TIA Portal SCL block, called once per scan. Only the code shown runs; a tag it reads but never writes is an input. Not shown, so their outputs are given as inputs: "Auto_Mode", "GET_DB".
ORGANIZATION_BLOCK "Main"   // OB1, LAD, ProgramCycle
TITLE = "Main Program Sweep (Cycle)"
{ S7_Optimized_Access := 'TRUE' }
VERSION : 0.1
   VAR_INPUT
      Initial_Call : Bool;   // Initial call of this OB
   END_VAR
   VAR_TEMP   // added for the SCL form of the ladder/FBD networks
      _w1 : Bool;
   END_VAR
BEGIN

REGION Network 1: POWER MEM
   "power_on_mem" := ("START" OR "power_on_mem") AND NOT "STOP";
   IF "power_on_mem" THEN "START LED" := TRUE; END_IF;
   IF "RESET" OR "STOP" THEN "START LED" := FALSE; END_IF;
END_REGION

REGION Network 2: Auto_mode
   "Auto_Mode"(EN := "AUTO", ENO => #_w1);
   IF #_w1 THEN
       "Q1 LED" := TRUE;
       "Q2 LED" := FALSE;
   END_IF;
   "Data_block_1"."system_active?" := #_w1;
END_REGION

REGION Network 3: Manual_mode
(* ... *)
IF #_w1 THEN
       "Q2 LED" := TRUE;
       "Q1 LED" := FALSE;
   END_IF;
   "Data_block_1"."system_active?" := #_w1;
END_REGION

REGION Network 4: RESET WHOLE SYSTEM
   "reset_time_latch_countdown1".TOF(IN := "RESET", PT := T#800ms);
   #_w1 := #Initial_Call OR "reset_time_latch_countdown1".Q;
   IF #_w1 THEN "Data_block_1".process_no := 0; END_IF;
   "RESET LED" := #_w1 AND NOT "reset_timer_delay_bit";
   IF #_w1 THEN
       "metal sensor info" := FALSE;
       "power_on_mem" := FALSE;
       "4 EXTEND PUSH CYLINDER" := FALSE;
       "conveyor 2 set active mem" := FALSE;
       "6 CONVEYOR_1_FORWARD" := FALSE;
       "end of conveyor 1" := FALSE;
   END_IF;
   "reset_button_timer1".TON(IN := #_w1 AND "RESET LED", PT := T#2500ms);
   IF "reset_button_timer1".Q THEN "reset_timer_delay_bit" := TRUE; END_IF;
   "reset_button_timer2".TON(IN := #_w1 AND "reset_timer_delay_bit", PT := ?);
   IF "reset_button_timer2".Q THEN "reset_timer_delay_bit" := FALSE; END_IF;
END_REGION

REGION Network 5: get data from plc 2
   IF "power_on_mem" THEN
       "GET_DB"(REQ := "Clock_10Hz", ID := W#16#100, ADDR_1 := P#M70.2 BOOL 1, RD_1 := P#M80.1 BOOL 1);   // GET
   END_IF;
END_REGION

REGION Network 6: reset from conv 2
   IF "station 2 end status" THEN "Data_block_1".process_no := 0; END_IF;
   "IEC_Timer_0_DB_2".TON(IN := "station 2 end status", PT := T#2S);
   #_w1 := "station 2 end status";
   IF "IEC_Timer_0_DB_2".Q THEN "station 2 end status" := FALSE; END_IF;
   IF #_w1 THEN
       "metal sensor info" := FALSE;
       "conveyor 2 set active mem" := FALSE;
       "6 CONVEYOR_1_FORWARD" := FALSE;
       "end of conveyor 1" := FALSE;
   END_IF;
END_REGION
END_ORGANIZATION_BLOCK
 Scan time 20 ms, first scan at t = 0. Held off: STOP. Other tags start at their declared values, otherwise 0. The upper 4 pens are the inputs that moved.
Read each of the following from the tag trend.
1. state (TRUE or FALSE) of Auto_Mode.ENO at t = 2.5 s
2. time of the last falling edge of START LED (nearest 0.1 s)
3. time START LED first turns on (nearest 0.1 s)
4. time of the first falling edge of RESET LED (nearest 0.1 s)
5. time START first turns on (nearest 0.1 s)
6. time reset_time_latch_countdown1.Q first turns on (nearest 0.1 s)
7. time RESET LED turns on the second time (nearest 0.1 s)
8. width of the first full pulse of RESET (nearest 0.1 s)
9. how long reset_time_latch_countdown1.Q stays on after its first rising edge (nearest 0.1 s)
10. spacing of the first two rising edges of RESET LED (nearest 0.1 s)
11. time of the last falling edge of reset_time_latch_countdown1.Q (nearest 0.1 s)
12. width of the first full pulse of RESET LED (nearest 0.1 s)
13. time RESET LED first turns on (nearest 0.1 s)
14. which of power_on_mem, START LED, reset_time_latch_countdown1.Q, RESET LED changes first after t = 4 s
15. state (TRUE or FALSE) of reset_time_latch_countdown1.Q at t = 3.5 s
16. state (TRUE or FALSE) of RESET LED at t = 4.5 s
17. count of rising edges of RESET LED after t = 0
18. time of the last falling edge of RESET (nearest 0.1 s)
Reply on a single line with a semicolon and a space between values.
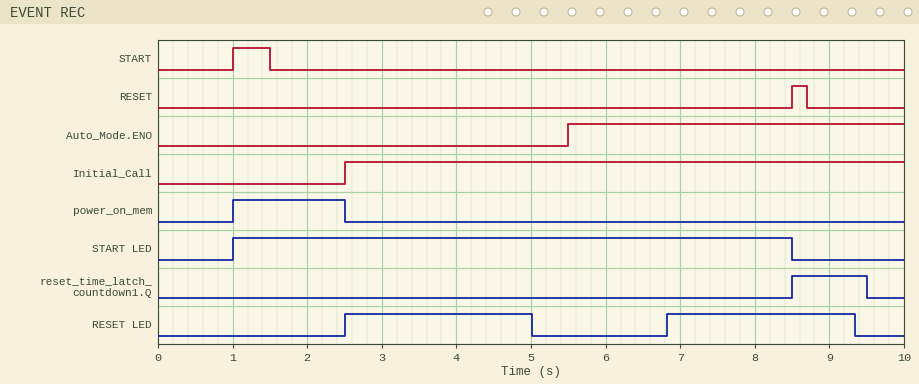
FALSE; 8.5 s; 1.0 s; 5.0 s; 1.0 s; 8.5 s; 6.8 s; 0.2 s; 1.0 s; 4.3 s; 9.5 s; 2.5 s; 2.5 s; RESET LED; FALSE; TRUE; 2; 8.7 s
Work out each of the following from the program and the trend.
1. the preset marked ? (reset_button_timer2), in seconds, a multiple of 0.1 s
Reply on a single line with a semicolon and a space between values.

1.8 s
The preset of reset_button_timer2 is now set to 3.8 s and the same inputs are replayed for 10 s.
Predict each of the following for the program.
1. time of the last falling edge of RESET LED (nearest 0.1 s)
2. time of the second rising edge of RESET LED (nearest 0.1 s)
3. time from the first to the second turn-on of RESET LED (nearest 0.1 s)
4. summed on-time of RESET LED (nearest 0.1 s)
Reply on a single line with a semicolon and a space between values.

5.0 s; 8.8 s; 6.3 s; 3.7 s
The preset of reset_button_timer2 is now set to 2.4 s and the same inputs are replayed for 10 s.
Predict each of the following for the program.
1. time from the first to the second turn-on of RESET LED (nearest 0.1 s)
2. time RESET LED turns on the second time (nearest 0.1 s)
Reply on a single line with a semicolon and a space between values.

4.9 s; 7.4 s
